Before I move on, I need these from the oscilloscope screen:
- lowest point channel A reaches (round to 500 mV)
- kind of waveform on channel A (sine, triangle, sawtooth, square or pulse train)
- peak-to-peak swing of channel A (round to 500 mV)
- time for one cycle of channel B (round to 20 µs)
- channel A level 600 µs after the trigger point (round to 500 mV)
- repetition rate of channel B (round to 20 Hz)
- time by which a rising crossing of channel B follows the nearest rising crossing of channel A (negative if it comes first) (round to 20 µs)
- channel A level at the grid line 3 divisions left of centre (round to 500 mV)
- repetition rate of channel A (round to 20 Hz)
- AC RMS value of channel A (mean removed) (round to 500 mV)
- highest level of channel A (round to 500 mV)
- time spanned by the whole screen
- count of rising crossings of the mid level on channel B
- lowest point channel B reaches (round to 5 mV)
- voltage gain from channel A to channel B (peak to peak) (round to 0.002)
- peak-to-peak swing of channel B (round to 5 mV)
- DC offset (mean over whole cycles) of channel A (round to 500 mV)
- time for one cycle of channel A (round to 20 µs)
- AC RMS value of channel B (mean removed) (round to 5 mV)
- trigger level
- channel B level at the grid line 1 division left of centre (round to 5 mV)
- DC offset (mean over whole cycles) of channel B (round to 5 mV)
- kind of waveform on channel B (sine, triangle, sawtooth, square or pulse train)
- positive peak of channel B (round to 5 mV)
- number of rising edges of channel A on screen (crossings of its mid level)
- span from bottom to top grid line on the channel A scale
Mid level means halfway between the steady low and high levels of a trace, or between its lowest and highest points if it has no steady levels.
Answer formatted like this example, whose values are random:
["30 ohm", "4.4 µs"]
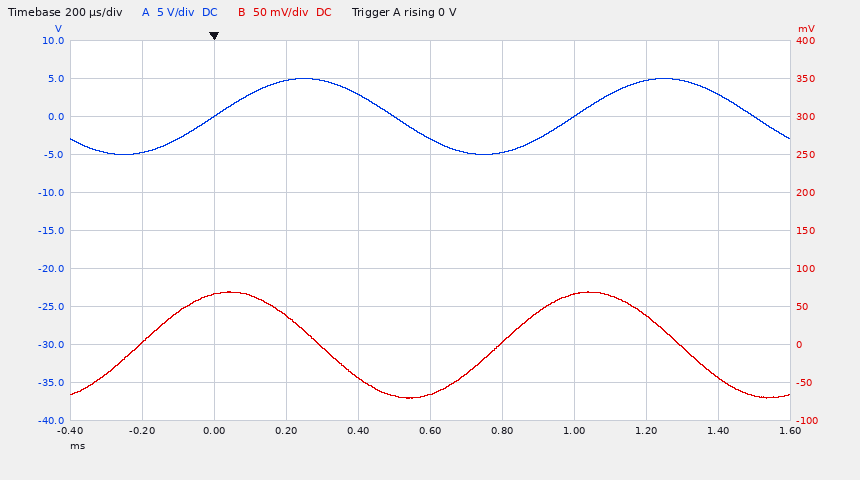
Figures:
["-5.0 V", "sine", "10.0 V", "1.00 ms", "-3.0 V", "1.00 kHz", "-200 µs", "0.0 V", "1.00 kHz", "3.5 V", "5.0 V", "2 ms", "2", "-70 mV", "0.014", "140 mV", "0.0 V", "1.00 ms", "50 mV", "0 V", "-45 mV", "0 mV", "sine", "70 mV", "2", "50 V"]
